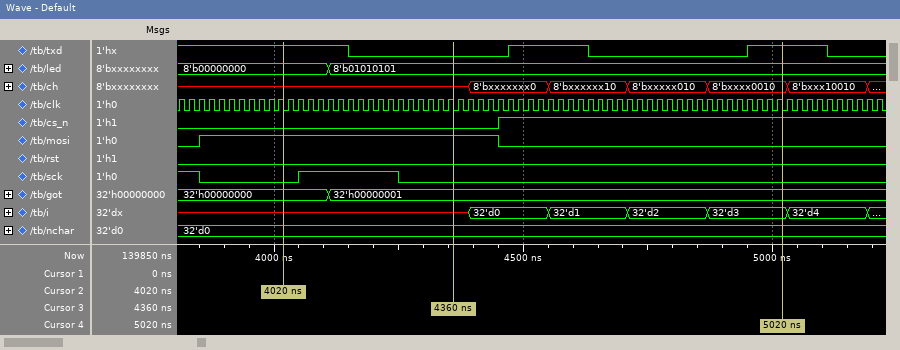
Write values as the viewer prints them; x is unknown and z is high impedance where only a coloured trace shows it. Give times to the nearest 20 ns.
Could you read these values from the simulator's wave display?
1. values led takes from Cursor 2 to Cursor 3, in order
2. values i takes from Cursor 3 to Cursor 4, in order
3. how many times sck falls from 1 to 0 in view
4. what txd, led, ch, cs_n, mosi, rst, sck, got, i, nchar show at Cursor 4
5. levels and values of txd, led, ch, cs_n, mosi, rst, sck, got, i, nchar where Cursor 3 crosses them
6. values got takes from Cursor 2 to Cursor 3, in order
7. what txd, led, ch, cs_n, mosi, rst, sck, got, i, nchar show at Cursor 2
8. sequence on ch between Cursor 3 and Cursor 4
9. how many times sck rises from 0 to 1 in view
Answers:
8'b00000000, 8'b01010101
x, 32'd0, 32'd1, 32'd2, 32'd3
2
txd=1, led=8'b01010101, ch=8'bxxxx0010, cs_n=1, mosi=0, rst=0, sck=0, got=32'h00000001, i=32'd3, nchar=32'd0
txd=0, led=8'b01010101, ch=x, cs_n=0, mosi=1, rst=0, sck=0, got=32'h00000001, i=x, nchar=32'd0
32'h00000000, 32'h00000001
txd=1, led=8'b00000000, ch=x, cs_n=0, mosi=1, rst=0, sck=0, got=32'h00000000, i=x, nchar=32'd0
x, 8'bxxxxxxx0, 8'bxxxxxx10, 8'bxxxxx010, 8'bxxxx0010
1
